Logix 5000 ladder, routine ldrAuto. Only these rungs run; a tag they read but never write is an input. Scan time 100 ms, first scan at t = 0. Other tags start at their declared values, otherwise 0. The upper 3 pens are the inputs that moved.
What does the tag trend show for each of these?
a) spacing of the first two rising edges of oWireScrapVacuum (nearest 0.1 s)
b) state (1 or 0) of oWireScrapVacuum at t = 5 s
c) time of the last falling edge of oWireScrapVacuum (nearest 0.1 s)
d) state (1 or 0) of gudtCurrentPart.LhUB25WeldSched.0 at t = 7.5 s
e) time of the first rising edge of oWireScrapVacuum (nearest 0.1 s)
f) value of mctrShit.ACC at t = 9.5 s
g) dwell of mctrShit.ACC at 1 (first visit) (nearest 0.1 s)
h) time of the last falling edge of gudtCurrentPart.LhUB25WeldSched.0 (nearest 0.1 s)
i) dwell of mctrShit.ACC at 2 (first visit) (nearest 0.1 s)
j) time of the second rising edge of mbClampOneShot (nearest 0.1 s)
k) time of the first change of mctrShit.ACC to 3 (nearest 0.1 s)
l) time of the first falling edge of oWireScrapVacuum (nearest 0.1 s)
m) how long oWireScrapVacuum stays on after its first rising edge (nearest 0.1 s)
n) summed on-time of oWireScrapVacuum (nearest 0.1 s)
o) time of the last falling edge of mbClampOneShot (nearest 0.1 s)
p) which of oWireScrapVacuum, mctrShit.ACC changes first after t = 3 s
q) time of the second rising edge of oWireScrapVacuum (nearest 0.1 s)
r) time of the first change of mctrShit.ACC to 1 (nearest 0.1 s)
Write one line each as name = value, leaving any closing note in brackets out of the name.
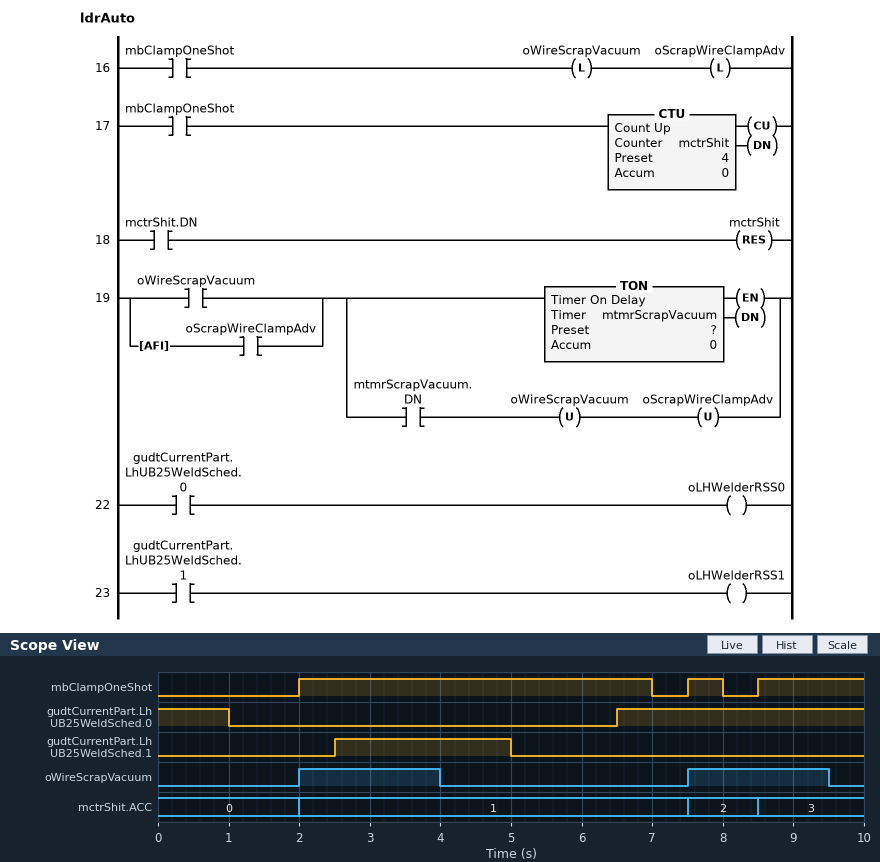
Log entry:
spacing of the first two rising edges of oWireScrapVacuum = 5.5 s
state (1 or 0) of oWireScrapVacuum at t = 5 s = 0
time of the last falling edge of oWireScrapVacuum = 9.5 s
state (1 or 0) of gudtCurrentPart.LhUB25WeldSched.0 at t = 7.5 s = 1
time of the first rising edge of oWireScrapVacuum = 2.0 s
value of mctrShit.ACC at t = 9.5 s = 3
dwell of mctrShit.ACC at 1 (first visit) = 5.5 s
time of the last falling edge of gudtCurrentPart.LhUB25WeldSched.0 = 1.0 s
dwell of mctrShit.ACC at 2 (first visit) = 1.0 s
time of the second rising edge of mbClampOneShot = 7.5 s
time of the first change of mctrShit.ACC to 3 = 8.5 s
time of the first falling edge of oWireScrapVacuum = 4.0 s
how long oWireScrapVacuum stays on after its first rising edge = 2.0 s
summed on-time of oWireScrapVacuum = 4.0 s
time of the last falling edge of mbClampOneShot = 8.0 s
which of oWireScrapVacuum, mctrShit.ACC changes first after t = 3 s = oWireScrapVacuum
time of the second rising edge of oWireScrapVacuum = 7.5 s
time of the first change of mctrShit.ACC to 1 = 2.0 s
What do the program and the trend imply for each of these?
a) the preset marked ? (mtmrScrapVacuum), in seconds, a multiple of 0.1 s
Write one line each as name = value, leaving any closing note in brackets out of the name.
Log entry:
the preset marked ? (mtmrScrapVacuum), in seconds, a multiple of 0.1 s = 2.0 s
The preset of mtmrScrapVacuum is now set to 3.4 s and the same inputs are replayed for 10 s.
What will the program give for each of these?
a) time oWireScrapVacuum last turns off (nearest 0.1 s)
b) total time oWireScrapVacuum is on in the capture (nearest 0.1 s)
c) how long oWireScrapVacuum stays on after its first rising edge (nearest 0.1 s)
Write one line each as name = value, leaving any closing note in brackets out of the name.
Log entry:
time oWireScrapVacuum last turns off = 5.4 s
total time oWireScrapVacuum is on in the capture = 5.9 s
how long oWireScrapVacuum stays on after its first rising edge = 3.4 s
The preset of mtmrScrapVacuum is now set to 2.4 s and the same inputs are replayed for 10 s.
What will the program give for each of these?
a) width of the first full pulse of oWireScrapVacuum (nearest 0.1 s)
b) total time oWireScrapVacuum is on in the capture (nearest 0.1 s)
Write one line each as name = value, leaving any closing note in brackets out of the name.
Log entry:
width of the first full pulse of oWireScrapVacuum = 2.4 s
total time oWireScrapVacuum is on in the capture = 4.8 s
